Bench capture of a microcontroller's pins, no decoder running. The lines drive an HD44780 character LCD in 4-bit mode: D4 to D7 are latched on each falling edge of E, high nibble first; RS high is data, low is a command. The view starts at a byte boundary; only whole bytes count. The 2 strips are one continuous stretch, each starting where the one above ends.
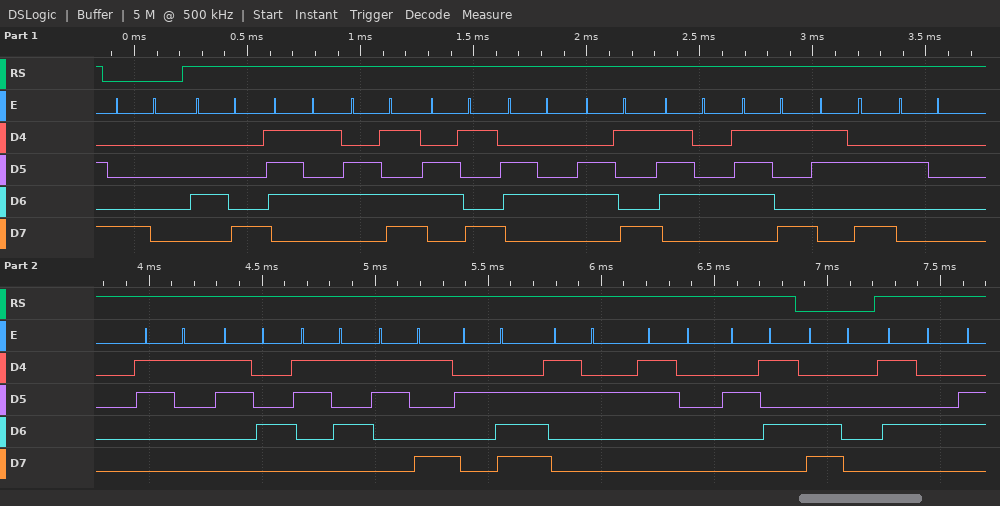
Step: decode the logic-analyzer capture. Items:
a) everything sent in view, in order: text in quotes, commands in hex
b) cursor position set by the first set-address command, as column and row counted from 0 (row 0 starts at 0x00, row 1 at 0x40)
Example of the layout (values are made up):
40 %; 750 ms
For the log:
0x80 "Humidity: 1459.20%" 0xC0 "T"; column 0, row 0
